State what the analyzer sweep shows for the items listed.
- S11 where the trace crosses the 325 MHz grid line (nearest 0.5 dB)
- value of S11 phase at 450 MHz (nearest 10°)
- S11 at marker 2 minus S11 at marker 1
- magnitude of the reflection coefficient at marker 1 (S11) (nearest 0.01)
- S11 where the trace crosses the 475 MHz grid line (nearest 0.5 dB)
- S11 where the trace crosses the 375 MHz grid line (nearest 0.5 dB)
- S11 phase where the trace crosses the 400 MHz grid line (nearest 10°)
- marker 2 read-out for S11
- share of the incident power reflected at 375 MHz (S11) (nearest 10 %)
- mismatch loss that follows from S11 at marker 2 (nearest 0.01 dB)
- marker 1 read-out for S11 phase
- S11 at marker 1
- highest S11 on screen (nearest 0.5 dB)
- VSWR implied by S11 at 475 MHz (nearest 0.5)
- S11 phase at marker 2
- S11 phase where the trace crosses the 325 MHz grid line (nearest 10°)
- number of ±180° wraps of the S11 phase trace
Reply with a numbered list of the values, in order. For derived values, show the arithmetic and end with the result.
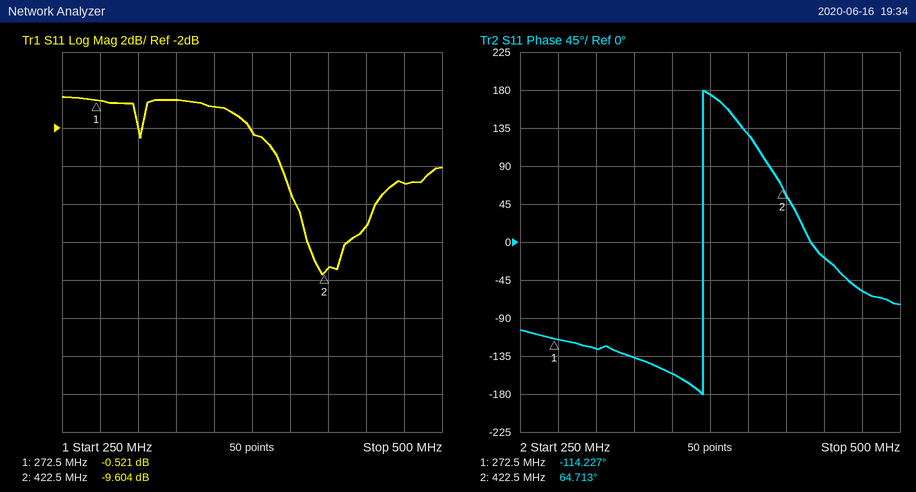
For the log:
1. -0.5 dB
2. -20°
3. -9.604 − (-0.521) = -9.083 dB
4. 10^(-0.521/20) ≈ 0.94
5. -5.0 dB
6. -2.0 dB
7. 130°
8. -9.604 dB
9. 10^(-2/10) ≈ 63.1 %, so 60 % to the nearest 10 %
10. −10 log10(1 − 10^(-9.604/10)) ≈ 0.50 dB
11. -114.227°
12. -0.521 dB
13. -0.5 dB
14. |Γ| = 10^(-5/20) = 0.5623; VSWR = (1 + 0.5623)/(1 − 0.5623) ≈ 3.57, so 3.5 to the nearest 0.5
15. 64.713°
16. -140°
17. 1
